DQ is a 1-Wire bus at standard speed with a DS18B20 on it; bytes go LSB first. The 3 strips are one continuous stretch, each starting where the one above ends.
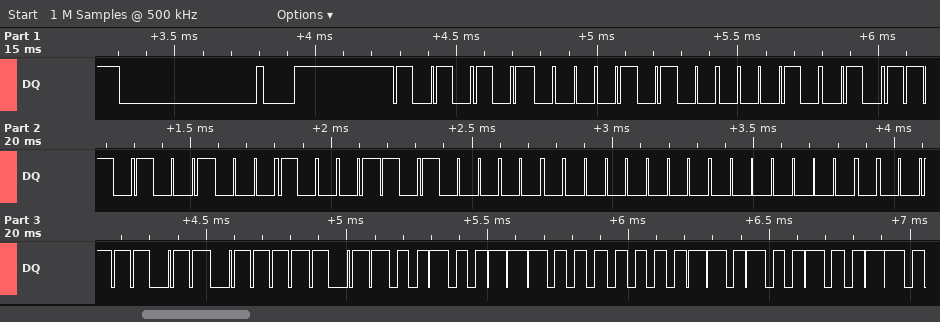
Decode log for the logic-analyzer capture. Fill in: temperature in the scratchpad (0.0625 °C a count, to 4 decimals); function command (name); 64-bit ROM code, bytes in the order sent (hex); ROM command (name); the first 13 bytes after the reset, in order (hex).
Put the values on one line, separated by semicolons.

28.5625 °C; Read Scratchpad; 28 48 97 88 05 00 00 DC; Match ROM; 55 28 48 97 88 05 00 00 DC BE C9 01 4B
